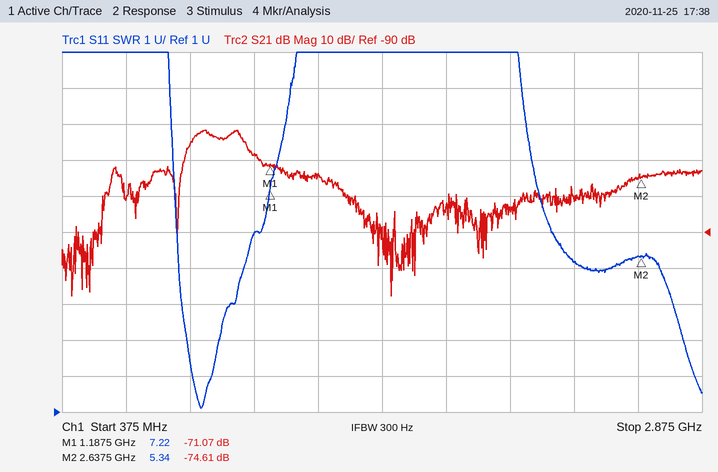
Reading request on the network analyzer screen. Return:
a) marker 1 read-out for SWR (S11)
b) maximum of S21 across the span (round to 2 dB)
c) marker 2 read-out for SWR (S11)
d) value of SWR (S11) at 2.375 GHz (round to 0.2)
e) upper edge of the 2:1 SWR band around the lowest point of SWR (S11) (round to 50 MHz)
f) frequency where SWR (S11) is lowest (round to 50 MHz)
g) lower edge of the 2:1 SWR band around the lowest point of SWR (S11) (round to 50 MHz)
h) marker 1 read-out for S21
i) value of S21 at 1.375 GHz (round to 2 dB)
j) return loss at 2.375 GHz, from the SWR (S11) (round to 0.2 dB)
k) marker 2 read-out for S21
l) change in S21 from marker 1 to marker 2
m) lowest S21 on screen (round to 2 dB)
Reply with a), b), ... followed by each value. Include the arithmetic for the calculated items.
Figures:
a) 7.22
b) -62 dB
c) 5.34
d) 5.2
e) 950 MHz
f) 900 MHz
g) 900 MHz
h) -71.07 dB
i) -74 dB
j) −20 log10((5.2 − 1)/(5.2 + 1)) ≈ 3.4 dB
k) -74.61 dB
l) -74.61 − (-71.07) = -3.54 dB
m) -108 dB
